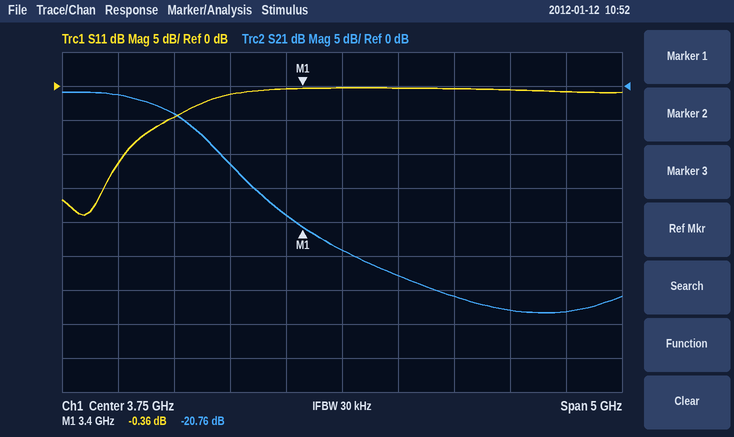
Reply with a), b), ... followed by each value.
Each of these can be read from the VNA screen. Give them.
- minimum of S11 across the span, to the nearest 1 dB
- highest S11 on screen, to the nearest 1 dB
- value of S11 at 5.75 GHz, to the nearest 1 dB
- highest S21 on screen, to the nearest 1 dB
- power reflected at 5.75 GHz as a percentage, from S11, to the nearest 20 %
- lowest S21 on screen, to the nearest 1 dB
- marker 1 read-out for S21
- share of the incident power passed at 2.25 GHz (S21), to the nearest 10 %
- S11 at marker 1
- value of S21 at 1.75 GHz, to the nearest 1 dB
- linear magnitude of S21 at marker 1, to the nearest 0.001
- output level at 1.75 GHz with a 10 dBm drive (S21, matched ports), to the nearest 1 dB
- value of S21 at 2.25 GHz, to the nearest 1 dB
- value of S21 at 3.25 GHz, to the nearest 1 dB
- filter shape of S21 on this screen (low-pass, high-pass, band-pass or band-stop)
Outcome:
a) -19 dB
b) 0 dB
c) -1 dB
d) -1 dB
e) 80 %
f) -33 dB
g) -20.76 dB
h) 40 %
i) -0.36 dB
j) -1 dB
k) 0.092
l) 9 dBm
m) -4 dB
n) -19 dB
o) low-pass
